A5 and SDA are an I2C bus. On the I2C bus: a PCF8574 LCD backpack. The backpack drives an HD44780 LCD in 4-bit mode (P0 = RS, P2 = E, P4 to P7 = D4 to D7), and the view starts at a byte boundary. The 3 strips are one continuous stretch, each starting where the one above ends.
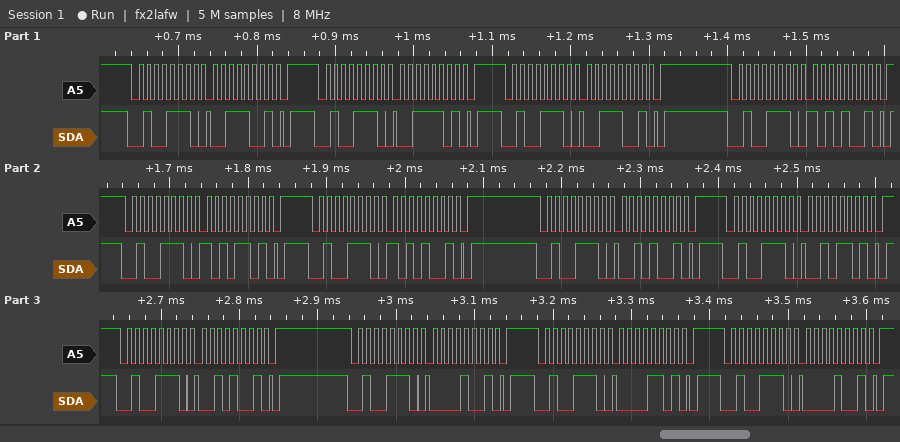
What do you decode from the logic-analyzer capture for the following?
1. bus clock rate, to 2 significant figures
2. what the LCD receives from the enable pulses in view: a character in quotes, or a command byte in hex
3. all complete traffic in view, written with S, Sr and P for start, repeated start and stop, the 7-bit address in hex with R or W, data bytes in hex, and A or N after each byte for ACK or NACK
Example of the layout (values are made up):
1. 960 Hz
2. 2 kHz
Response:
1. 100 kHz
2. ':' ' '
3. S 27W A 39 A P S 27W A 3D A P S 27W A 39 A P S 27W A A9 A P S 27W A AD A P S 27W A A9 A P S 27W A 29 A P S 27W A 2D A P S 27W A 29 A P S 27W A 09 A P S 27W A 0D A P S 27W A 09 A P
